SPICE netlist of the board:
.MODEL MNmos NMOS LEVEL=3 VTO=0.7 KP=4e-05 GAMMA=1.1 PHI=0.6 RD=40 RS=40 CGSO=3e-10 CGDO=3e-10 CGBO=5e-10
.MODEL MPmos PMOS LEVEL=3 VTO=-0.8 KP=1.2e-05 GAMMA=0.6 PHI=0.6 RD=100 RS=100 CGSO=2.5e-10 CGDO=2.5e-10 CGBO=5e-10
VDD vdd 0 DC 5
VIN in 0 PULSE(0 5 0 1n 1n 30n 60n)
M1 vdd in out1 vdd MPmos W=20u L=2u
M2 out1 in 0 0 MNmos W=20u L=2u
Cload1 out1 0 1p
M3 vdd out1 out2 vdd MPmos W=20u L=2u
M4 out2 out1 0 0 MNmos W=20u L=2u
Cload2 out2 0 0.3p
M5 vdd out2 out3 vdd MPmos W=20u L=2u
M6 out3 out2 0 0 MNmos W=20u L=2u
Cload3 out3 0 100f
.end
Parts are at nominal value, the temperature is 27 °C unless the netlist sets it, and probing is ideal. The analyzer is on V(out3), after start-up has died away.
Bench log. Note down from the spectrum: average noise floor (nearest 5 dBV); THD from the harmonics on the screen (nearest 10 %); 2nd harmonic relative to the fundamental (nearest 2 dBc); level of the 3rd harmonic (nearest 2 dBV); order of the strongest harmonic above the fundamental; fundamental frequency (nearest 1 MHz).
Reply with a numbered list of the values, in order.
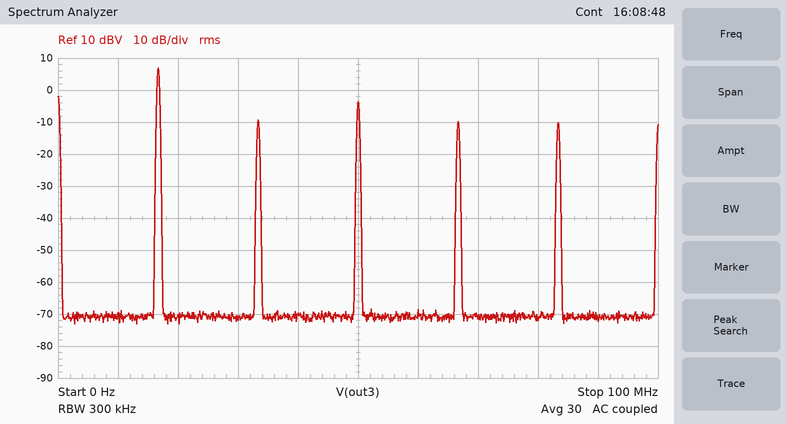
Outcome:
1. -70 dBV
2. 40 %
3. -16 dBc
4. -4 dBV
5. 3
6. 17 MHz
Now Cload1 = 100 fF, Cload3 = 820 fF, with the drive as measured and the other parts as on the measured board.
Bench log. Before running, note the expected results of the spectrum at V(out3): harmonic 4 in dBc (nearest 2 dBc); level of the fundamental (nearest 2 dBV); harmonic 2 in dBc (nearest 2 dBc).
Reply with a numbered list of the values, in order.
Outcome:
1. -20 dBc
2. 6 dBV
3. -18 dBc
